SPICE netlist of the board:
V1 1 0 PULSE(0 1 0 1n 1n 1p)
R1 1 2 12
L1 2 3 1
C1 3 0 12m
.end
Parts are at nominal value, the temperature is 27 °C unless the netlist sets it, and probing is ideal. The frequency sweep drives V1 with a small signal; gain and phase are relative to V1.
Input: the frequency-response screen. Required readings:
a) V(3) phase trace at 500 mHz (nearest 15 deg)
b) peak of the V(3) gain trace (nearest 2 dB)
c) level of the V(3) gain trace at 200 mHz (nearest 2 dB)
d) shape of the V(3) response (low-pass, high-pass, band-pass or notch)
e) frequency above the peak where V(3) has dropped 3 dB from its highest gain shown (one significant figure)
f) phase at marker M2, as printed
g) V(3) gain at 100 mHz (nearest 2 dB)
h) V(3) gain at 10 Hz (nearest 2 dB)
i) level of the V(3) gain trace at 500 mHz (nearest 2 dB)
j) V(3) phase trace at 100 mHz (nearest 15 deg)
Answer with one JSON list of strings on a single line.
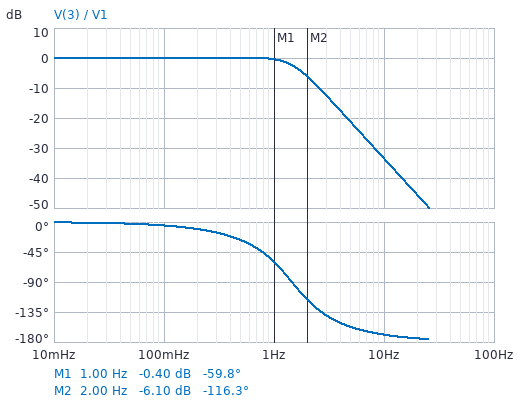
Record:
["-30 deg", "0 dB", "0 dB", "low-pass", "2 Hz", "-116.3 deg", "0 dB", "-34 dB", "0 dB", "0 deg"]
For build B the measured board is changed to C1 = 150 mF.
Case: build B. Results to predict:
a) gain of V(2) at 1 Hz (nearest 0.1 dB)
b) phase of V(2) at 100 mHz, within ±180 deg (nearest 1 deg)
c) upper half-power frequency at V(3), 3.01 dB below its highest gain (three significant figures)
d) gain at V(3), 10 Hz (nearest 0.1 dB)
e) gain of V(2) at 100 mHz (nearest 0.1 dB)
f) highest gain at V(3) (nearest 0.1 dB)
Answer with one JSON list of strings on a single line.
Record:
["-8.0 dB", "-50 deg", "92.7 mHz", "-55.6 dB", "-3.9 dB", "0 dB"]
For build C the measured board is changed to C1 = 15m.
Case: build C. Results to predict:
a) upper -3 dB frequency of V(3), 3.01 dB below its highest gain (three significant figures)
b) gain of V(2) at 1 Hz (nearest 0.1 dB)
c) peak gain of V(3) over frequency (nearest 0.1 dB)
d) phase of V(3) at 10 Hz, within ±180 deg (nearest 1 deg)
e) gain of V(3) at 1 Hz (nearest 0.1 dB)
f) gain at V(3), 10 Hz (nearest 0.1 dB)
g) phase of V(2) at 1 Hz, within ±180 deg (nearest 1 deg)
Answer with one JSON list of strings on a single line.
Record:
["1.25 Hz", "-9.4 dB", "0 dB", "-169 deg", "-1.6 dB", "-35.5 dB", "-70 deg"]
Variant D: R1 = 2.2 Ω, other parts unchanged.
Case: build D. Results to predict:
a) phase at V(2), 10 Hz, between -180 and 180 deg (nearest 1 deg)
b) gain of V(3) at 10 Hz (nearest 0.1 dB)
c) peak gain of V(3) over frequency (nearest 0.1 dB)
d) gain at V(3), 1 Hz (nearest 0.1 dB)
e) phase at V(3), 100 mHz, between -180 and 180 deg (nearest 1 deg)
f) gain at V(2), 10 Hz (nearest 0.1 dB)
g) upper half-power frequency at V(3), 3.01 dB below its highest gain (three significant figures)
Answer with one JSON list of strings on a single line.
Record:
["2 deg", "-33.3 dB", "12.4 dB", "5.2 dB", "-1 deg", "0 dB", "1.60 Hz"]
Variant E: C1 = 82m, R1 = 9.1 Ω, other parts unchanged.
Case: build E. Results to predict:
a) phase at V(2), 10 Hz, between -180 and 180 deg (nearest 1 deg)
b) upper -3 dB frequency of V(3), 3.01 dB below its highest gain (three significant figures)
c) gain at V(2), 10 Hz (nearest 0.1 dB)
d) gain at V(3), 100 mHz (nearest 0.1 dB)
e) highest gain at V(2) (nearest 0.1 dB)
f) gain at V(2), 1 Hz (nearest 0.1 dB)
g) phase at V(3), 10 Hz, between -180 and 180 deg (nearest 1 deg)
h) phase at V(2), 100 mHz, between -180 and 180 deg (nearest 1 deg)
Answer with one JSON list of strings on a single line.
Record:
["8 deg", "249 mHz", "-0.1 dB", "-0.6 dB", "0 dB", "-7.3 dB", "-172 deg", "-26 deg"]
